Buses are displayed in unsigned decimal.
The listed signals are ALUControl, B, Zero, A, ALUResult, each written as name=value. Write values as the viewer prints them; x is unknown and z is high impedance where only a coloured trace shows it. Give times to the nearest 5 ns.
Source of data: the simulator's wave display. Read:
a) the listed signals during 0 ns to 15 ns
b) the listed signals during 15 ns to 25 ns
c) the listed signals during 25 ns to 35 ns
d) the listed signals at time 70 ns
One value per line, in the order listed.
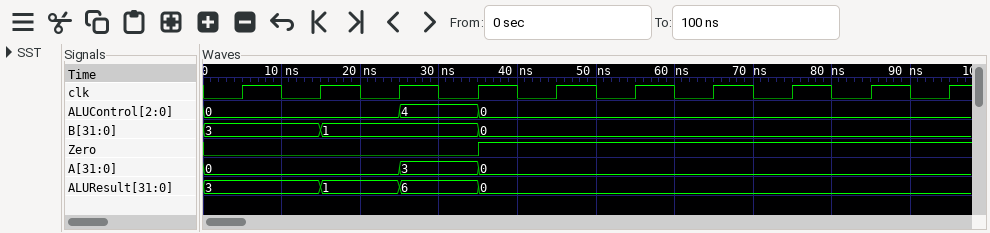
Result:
ALUControl=0, B=3, Zero=0, A=0, ALUResult=3
ALUControl=0, B=1, Zero=0, A=0, ALUResult=1
ALUControl=4, B=1, Zero=0, A=3, ALUResult=6
ALUControl=0, B=0, Zero=1, A=0, ALUResult=0
